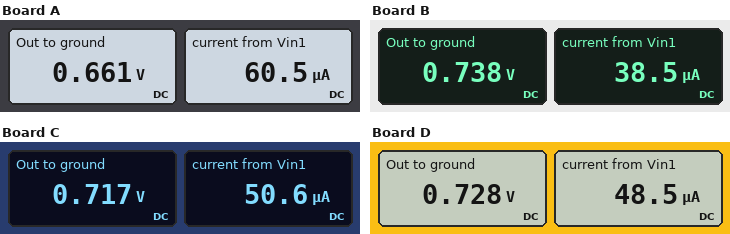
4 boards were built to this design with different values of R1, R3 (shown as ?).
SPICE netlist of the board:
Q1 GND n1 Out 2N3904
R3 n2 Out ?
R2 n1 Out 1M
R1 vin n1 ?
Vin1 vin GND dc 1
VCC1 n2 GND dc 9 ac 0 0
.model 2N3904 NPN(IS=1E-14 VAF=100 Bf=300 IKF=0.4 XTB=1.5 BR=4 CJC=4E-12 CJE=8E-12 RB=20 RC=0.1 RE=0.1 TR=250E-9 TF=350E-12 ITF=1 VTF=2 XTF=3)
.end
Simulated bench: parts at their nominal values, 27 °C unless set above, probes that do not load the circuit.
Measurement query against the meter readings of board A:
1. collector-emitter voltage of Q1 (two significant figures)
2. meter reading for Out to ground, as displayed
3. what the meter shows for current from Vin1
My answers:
-660 mV
0.661 V
60.5 µA
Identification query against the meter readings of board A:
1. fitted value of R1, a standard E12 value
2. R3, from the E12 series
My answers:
5.6 kΩ
6.8 kΩ
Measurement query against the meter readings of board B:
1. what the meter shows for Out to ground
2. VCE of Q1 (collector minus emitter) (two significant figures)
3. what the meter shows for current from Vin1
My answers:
0.738 V
-740 mV
38.5 µA
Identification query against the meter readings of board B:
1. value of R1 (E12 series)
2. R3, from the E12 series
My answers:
6.8 kΩ
1 kΩ
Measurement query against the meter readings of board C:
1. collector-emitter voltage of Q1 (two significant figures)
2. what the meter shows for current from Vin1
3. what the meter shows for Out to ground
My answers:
-720 mV
50.6 µA
0.717 V
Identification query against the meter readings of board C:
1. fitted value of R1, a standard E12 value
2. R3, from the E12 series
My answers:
5.6 kΩ
1.5 kΩ
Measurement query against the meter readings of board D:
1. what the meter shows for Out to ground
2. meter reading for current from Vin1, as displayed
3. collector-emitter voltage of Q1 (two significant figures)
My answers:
0.728 V
48.5 µA
-730 mV
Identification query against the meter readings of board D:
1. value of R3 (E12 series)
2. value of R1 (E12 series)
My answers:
1.2 kΩ
5.6 kΩ
